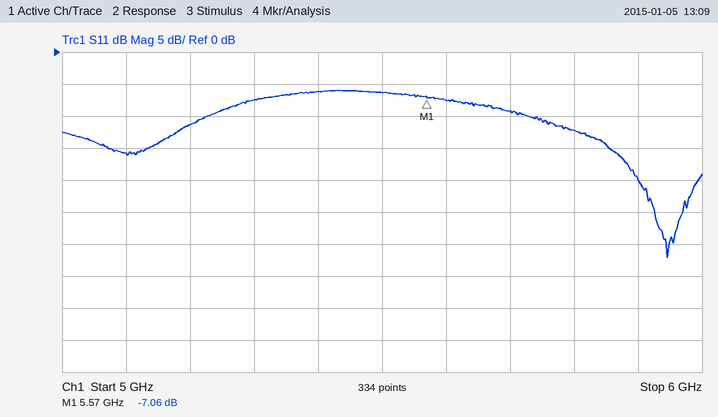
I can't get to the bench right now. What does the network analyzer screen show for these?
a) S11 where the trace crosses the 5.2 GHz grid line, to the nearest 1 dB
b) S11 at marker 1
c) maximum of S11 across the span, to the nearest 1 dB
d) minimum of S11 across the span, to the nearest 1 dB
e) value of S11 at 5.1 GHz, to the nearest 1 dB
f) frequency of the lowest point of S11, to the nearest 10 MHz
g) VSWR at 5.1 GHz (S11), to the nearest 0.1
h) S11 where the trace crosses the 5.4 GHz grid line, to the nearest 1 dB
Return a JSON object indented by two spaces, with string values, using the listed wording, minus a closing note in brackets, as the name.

{
  "S11 where the trace crosses the 5.2 GHz grid line, to the nearest 1 dB": "-11 dB",
  "S11 at marker 1": "-7.06 dB",
  "maximum of S11 across the span, to the nearest 1 dB": "-6 dB",
  "minimum of S11 across the span, to the nearest 1 dB": "-32 dB",
  "value of S11 at 5.1 GHz, to the nearest 1 dB": "-16 dB",
  "frequency of the lowest point of S11, to the nearest 10 MHz": "5.95 GHz",
  "VSWR at 5.1 GHz (S11), to the nearest 0.1": "1.4",
  "S11 where the trace crosses the 5.4 GHz grid line, to the nearest 1 dB": "-6 dB"
}
